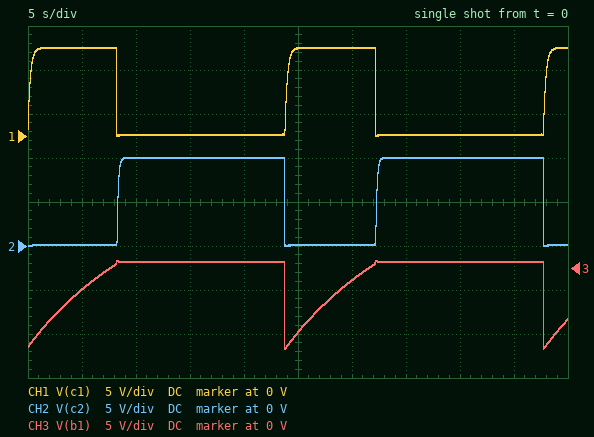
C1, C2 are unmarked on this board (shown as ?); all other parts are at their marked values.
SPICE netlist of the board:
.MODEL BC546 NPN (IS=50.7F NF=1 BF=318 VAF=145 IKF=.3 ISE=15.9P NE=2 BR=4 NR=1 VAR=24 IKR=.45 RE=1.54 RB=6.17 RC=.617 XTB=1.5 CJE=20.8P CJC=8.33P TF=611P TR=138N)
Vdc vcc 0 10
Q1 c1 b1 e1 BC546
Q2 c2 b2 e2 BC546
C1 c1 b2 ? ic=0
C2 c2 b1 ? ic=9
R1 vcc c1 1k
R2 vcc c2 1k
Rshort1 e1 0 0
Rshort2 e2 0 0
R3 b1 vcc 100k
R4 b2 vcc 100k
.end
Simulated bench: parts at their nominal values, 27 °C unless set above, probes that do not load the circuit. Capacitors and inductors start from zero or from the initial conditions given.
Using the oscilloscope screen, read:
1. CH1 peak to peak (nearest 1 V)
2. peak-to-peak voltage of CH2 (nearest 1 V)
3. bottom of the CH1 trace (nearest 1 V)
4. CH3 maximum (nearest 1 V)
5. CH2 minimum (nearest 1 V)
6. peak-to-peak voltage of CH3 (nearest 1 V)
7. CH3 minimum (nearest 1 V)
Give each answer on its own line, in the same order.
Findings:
10 V
10 V
0 V
1 V
0 V
10 V
-9 V
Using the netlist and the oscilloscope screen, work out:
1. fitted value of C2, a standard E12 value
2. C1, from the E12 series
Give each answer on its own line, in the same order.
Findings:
120 µF
220 µF
